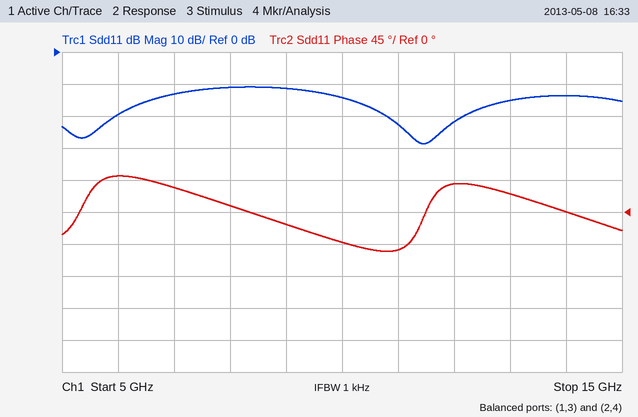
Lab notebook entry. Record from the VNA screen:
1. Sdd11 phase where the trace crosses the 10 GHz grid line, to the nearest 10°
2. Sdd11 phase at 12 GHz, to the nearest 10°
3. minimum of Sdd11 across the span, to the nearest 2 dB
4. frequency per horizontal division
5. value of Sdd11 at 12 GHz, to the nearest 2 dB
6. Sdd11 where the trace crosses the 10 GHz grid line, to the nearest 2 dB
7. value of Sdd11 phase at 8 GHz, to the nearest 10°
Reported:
-40°
40°
-28 dB
1 GHz
-22 dB
-14 dB
10°
